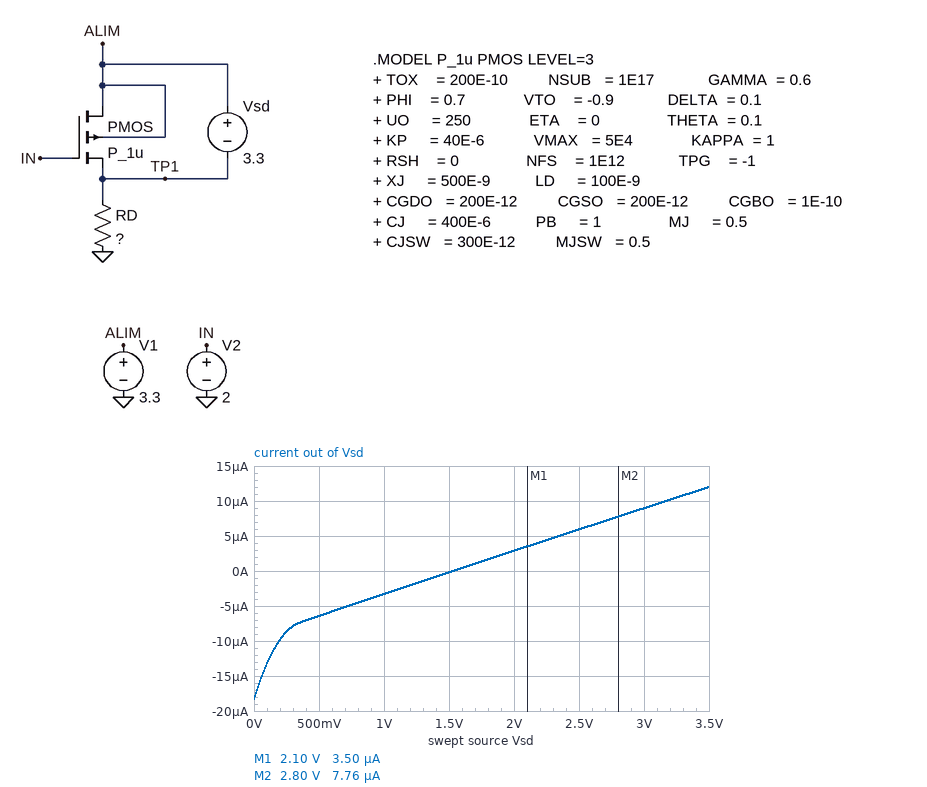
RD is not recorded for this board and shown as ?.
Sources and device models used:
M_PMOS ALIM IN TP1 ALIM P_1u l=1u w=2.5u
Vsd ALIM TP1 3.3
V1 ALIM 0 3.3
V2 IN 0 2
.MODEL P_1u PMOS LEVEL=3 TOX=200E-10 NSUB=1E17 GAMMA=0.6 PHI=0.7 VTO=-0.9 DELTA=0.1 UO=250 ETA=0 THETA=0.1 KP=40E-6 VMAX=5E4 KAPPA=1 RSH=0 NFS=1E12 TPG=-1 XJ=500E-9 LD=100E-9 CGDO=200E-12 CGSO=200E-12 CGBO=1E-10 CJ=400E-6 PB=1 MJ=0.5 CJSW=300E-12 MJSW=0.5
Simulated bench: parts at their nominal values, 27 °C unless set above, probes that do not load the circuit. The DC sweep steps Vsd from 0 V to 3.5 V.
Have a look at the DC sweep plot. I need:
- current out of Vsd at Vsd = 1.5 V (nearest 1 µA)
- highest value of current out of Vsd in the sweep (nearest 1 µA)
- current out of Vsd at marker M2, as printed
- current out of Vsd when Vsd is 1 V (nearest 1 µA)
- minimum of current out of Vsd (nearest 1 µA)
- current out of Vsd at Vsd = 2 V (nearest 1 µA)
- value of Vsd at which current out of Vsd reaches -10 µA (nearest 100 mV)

0 A
12 µA
7.76 µA
-3 µA
-18 µA
3 µA
200 mV
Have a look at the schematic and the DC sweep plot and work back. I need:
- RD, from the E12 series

180 kΩ
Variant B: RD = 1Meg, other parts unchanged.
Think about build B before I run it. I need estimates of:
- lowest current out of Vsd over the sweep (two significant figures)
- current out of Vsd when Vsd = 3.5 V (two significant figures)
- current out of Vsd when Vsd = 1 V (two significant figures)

-3.3 µA
11 µA
7.2 µA
